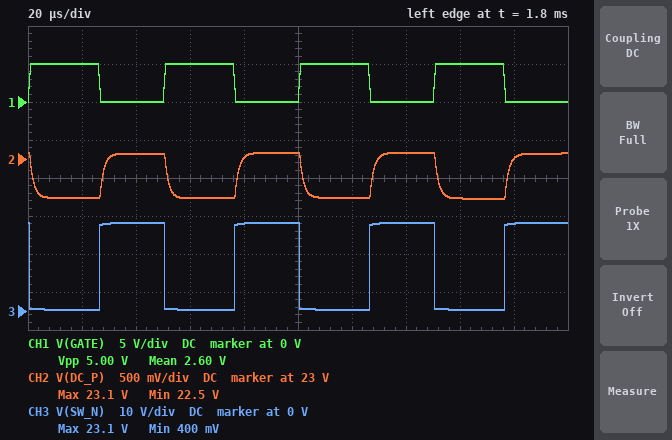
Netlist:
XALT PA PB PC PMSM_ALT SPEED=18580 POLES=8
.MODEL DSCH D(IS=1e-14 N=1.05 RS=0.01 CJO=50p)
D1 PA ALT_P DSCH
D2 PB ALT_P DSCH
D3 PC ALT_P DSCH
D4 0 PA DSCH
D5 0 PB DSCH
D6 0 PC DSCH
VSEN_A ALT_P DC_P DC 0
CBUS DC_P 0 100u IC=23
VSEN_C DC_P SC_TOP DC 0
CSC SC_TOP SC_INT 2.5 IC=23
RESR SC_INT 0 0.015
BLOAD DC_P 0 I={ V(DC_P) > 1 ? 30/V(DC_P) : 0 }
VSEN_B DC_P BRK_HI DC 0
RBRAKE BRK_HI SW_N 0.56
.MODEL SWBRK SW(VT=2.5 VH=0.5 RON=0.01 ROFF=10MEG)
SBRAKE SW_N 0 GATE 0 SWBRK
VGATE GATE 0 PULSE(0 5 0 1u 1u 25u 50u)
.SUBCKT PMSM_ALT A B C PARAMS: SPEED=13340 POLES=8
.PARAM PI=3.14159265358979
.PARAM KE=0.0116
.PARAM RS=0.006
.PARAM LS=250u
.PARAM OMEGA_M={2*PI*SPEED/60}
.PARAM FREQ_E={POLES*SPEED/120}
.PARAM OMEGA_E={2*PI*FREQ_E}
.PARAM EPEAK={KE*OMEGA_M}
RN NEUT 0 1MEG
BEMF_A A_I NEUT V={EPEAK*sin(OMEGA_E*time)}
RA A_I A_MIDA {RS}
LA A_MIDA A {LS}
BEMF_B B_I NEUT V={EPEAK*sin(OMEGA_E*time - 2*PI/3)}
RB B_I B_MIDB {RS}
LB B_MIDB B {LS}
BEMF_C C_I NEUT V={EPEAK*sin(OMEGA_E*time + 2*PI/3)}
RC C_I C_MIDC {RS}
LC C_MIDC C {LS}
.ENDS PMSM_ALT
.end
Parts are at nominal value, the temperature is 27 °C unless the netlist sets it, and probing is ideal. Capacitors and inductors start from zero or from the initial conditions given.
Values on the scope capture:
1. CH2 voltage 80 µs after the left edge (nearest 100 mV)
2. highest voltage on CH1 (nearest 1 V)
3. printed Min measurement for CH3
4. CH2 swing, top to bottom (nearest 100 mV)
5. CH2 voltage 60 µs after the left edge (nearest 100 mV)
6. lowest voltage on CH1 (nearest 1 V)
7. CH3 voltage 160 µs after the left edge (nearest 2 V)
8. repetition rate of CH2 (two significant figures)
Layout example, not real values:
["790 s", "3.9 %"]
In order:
["23.0 V", "5 V", "400 mV", "600 mV", "22.5 V", "0 V", "0 V", "20 kHz"]
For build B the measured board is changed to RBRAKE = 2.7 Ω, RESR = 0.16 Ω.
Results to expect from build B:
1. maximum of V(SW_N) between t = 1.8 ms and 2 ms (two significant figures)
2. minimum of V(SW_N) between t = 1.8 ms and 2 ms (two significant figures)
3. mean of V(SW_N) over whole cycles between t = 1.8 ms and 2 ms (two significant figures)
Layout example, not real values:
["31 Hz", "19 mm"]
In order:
["24 V", "84 mV", "11 V"]
